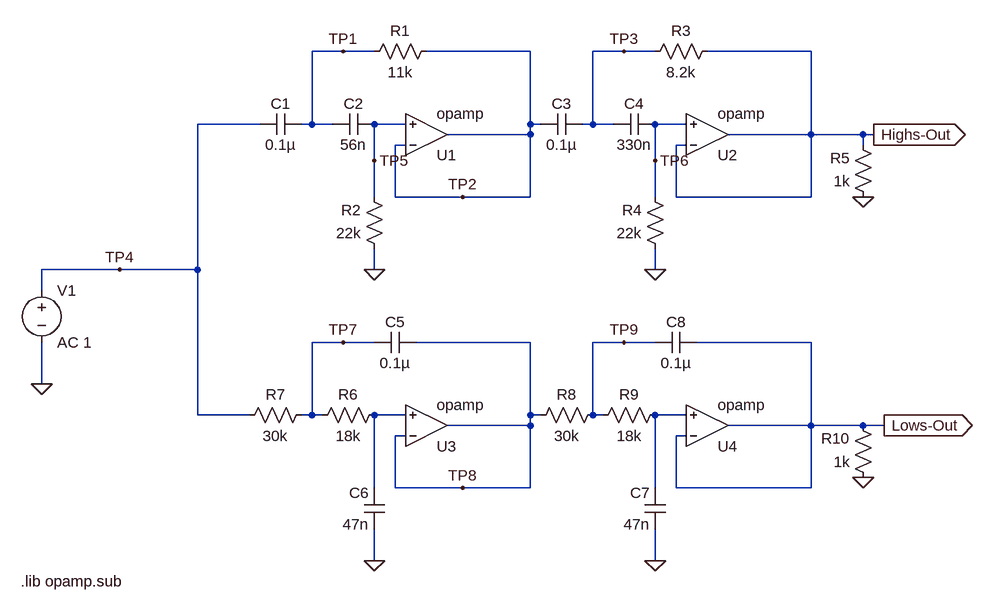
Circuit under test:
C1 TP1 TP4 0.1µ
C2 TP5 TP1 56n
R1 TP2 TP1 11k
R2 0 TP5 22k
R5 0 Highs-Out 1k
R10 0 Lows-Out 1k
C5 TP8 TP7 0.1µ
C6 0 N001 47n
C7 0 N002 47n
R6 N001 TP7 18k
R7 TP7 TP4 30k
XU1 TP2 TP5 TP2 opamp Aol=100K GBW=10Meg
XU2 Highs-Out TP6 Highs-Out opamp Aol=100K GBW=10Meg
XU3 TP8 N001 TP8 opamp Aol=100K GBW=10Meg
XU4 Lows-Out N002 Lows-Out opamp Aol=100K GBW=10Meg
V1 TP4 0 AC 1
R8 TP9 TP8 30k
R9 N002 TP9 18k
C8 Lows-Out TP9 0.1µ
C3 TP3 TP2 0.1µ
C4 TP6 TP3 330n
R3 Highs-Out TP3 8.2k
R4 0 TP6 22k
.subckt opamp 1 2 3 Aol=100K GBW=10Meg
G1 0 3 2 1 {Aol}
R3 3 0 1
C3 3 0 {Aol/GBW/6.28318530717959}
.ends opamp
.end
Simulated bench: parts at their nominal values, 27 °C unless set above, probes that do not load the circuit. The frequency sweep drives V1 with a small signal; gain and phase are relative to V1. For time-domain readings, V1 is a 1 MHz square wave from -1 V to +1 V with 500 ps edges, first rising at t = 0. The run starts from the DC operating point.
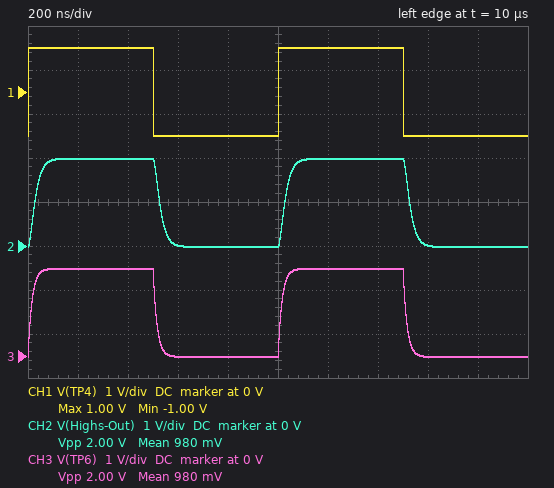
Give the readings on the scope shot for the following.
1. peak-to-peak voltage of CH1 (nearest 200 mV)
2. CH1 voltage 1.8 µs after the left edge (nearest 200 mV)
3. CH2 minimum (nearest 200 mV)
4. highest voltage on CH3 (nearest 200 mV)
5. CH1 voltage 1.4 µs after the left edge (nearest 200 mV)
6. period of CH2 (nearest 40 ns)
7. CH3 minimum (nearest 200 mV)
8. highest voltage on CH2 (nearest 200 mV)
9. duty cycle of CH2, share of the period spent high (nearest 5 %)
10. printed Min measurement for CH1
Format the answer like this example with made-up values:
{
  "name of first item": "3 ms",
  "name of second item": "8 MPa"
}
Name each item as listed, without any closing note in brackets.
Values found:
{
  "peak-to-peak voltage of CH1": "2.0 V",
  "CH1 voltage 1.8 µs after the left edge": "-1.0 V",
  "CH2 minimum": "0 V",
  "highest voltage on CH3": "2.0 V",
  "CH1 voltage 1.4 µs after the left edge": "1.0 V",
  "period of CH2": "1.00 µs",
  "CH3 minimum": "0 V",
  "highest voltage on CH2": "2.0 V",
  "duty cycle of CH2, share of the period spent high": "50 %",
  "printed Min measurement for CH1": "-1.00 V"
}
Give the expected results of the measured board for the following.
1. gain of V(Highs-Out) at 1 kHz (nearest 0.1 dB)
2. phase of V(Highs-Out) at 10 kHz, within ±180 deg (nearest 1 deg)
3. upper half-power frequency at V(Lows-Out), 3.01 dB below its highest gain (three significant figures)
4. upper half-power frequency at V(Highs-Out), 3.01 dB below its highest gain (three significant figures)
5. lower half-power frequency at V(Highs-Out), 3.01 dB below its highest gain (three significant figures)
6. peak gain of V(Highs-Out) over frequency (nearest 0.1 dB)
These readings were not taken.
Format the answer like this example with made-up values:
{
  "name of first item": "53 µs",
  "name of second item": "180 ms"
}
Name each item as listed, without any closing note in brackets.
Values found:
{
  "gain of V(Highs-Out) at 1 kHz": "0 dB",
  "phase of V(Highs-Out) at 10 kHz, within ±180 deg": "2 deg",
  "upper half-power frequency at V(Lows-Out), 3.01 dB below its highest gain": "80.0 Hz",
  "upper half-power frequency at V(Highs-Out), 3.01 dB below its highest gain": "6.44 MHz",
  "lower half-power frequency at V(Highs-Out), 3.01 dB below its highest gain": "147 Hz",
  "peak gain of V(Highs-Out) over frequency": "0 dB"
}
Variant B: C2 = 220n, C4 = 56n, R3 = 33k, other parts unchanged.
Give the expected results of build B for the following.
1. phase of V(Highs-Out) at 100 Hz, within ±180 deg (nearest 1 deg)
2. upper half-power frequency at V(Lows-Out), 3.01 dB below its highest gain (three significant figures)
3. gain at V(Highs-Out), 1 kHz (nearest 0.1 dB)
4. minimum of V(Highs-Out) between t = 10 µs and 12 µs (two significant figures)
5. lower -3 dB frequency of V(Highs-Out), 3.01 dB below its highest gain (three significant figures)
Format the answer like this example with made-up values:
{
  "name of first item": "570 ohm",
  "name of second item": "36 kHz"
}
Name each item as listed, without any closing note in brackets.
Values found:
{
  "phase of V(Highs-Out) at 100 Hz, within ±180 deg": "143 deg",
  "upper half-power frequency at V(Lows-Out), 3.01 dB below its highest gain": "80.0 Hz",
  "gain at V(Highs-Out), 1 kHz": "-0.1 dB",
  "minimum of V(Highs-Out) between t = 10 µs and 12 µs": "-23 mV",
  "lower -3 dB frequency of V(Highs-Out), 3.01 dB below its highest gain": "183 Hz"
}
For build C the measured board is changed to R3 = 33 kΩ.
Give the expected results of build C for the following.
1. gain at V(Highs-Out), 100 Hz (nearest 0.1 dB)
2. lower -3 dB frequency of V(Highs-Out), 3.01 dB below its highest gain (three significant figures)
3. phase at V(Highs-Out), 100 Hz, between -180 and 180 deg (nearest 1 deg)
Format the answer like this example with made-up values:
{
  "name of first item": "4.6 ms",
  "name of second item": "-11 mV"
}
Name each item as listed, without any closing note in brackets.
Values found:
{
  "gain at V(Highs-Out), 100 Hz": "-9.1 dB",
  "lower -3 dB frequency of V(Highs-Out), 3.01 dB below its highest gain": "164 Hz",
  "phase at V(Highs-Out), 100 Hz, between -180 and 180 deg": "160 deg"
}
